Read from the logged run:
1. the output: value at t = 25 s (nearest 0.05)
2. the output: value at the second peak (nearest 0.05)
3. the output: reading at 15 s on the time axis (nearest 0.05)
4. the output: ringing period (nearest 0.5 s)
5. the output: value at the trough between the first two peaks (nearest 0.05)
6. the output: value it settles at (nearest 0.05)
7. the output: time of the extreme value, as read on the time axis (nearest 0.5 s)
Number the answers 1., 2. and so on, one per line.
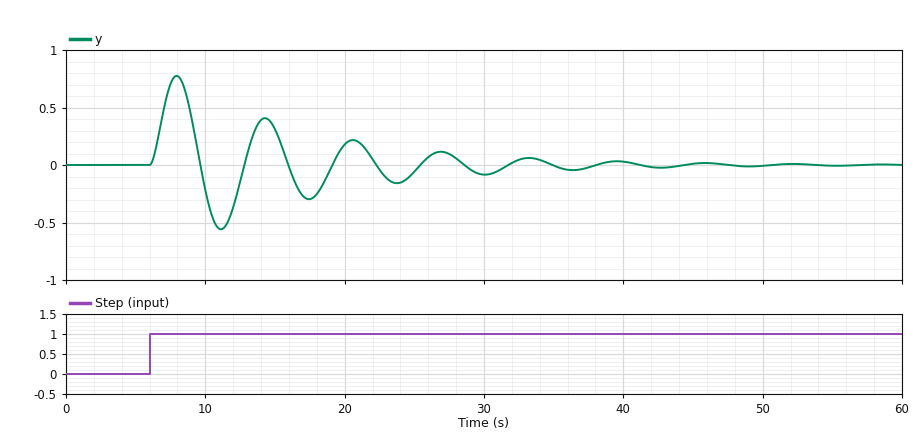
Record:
1. -0.05
2. 0.40
3. 0.30
4. 6.5 s
5. -0.55
6. 0.00
7. 8.0 s
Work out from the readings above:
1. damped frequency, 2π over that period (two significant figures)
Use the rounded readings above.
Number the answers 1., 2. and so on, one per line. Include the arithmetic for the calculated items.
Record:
1. 2π / 6.5 = 0.97 rad/s
